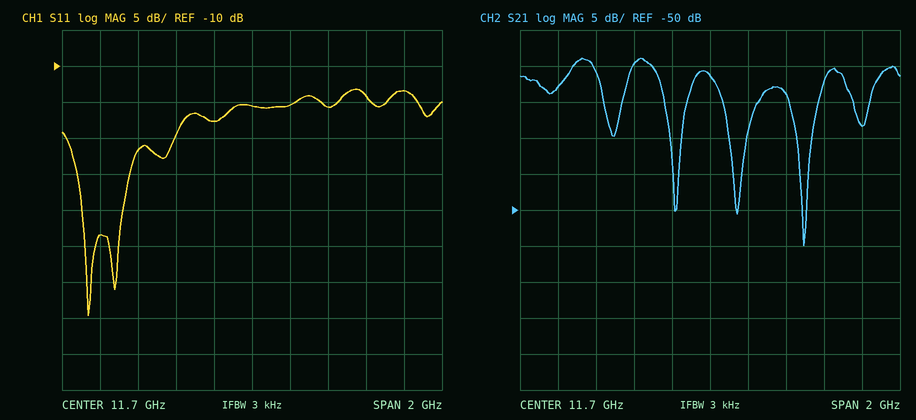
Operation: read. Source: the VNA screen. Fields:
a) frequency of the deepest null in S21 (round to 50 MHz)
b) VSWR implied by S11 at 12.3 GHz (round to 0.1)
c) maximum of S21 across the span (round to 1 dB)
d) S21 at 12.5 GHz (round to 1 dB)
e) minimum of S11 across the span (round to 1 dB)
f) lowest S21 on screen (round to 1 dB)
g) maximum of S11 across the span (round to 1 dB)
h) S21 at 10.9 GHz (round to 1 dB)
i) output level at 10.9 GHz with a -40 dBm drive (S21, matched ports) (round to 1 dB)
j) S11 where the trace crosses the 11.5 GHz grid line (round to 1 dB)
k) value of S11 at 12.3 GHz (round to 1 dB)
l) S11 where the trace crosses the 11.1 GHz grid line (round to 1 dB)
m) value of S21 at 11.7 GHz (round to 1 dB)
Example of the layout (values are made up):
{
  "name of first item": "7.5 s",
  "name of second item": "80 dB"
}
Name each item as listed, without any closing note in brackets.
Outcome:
{
  "frequency of the deepest null in S21": "12.20 GHz",
  "VSWR implied by S11 at 12.3 GHz": "1.5",
  "maximum of S21 across the span": "-29 dB",
  "S21 at 12.5 GHz": "-38 dB",
  "minimum of S11 across the span": "-45 dB",
  "lowest S21 on screen": "-55 dB",
  "maximum of S11 across the span": "-13 dB",
  "S21 at 10.9 GHz": "-33 dB",
  "output level at 10.9 GHz with a -40 dBm drive (S21, matched ports)": "-73 dBm",
  "S11 where the trace crosses the 11.5 GHz grid line": "-18 dB",
  "value of S11 at 12.3 GHz": "-14 dB",
  "S11 where the trace crosses the 11.1 GHz grid line": "-22 dB",
  "value of S21 at 11.7 GHz": "-31 dB"
}
